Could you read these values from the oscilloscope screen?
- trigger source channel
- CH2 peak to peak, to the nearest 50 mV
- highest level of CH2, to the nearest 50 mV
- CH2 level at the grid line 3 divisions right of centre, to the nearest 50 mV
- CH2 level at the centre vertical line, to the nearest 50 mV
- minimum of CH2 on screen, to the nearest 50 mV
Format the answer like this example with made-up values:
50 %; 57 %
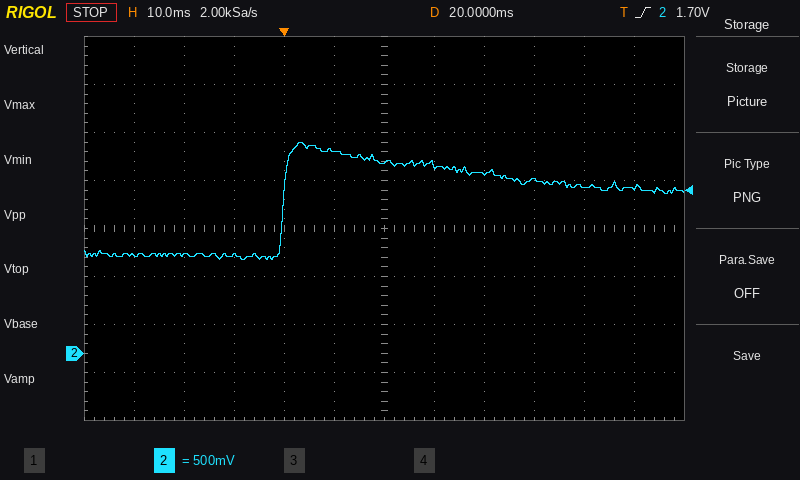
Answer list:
CH2; 1.20 V; 2.20 V; 1.80 V; 2.00 V; 1.00 V
